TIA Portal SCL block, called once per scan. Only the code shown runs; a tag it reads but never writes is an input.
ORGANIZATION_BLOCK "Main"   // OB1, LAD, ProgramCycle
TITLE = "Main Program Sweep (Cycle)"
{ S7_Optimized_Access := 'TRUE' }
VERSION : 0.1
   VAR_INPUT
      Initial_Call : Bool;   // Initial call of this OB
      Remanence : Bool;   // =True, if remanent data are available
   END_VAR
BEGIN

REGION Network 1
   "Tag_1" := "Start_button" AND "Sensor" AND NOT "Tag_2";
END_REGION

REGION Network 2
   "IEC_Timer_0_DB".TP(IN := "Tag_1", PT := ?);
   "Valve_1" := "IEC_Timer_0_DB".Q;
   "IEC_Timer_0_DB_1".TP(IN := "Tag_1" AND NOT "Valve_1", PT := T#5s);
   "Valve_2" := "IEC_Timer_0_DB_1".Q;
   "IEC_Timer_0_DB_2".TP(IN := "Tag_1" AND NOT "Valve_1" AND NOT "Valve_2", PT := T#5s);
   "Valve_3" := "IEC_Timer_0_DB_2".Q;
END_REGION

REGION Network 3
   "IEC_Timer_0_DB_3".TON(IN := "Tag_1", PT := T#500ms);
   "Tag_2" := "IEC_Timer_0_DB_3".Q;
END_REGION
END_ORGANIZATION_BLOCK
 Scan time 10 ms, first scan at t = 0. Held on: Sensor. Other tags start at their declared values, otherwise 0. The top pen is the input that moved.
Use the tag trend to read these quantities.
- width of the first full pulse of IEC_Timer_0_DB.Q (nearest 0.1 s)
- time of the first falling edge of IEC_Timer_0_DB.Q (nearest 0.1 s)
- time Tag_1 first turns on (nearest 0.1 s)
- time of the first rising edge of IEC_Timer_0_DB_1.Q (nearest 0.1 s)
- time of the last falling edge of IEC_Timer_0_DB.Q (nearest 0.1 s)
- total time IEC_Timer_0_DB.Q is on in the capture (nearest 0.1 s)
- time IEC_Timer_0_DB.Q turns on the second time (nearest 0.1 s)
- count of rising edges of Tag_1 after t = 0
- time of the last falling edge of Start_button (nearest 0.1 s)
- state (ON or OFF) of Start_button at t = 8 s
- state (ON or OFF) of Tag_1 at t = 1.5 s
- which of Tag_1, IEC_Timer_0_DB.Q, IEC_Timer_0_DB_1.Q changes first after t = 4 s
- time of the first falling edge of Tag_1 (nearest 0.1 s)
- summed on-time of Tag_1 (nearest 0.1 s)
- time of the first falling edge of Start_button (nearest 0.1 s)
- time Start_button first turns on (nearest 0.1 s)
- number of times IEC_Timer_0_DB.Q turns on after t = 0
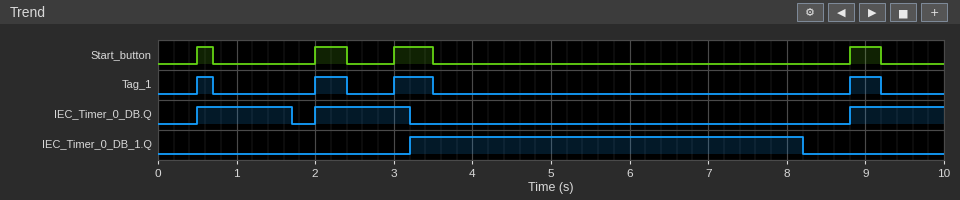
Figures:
1.2 s
1.7 s
0.5 s
3.2 s
3.2 s
3.6 s
2.0 s
4
9.2 s
OFF
OFF
IEC_Timer_0_DB_1.Q
0.7 s
1.5 s
0.7 s
0.5 s
3
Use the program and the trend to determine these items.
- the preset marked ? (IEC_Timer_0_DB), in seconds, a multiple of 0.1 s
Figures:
1.2 s
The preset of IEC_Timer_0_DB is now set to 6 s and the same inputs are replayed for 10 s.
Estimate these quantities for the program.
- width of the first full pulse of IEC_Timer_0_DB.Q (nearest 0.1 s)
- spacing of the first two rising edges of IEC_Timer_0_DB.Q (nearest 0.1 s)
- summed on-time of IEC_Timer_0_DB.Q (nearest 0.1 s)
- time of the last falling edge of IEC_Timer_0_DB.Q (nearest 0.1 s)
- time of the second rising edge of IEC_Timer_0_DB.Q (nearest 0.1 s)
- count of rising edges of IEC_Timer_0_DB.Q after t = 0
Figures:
6.0 s
8.3 s
7.2 s
6.5 s
8.8 s
2
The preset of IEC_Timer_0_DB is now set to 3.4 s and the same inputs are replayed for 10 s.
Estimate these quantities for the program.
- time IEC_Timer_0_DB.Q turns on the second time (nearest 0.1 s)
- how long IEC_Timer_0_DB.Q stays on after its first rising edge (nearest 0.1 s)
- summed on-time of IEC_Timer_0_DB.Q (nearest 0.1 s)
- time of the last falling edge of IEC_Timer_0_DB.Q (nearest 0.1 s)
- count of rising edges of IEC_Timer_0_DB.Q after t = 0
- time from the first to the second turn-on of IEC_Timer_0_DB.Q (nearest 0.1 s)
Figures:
8.8 s
3.4 s
4.6 s
3.9 s
2
8.3 s
